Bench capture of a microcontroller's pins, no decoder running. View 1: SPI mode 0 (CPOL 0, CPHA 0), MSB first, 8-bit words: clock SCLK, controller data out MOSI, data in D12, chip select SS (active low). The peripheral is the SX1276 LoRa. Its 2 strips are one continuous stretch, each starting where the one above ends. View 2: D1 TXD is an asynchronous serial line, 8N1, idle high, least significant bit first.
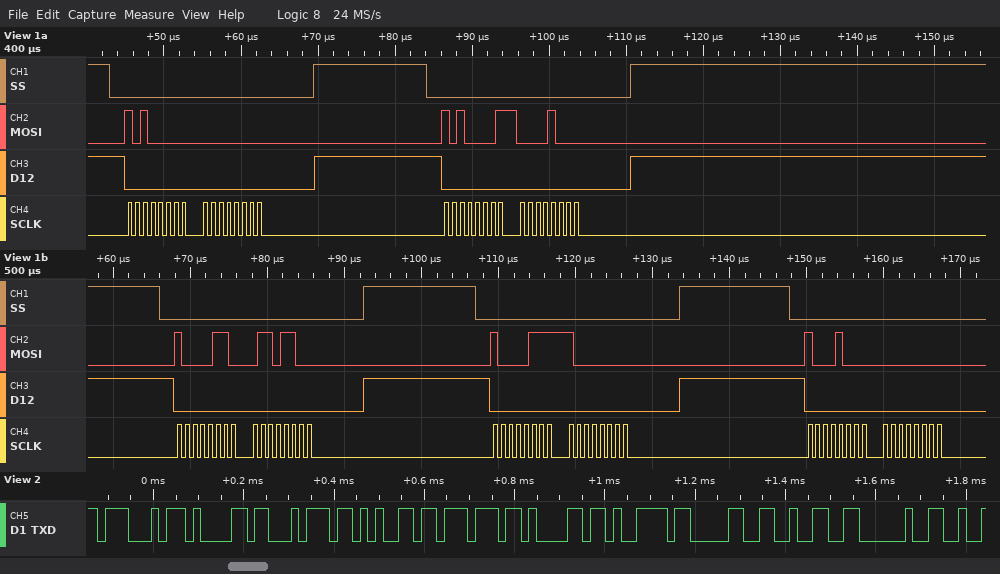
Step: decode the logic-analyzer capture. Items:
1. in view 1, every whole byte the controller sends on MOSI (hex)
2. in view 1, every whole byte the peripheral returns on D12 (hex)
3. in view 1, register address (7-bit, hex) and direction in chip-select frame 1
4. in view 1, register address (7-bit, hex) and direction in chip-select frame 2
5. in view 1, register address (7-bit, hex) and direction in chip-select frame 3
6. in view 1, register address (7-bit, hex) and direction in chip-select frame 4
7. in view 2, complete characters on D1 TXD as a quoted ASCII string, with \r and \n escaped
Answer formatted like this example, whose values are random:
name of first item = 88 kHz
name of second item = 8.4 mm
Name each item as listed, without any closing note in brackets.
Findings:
in view 1, every whole byte the controller sends on MOSI = 0xA0 0x00 0xA1 0x08 0x86 0x6C 0x87 0x80 0x88 0x00
in view 1, every whole byte the peripheral returns on D12 = 0x00 0x00 0x00 0x00 0x00 0x00 0x00 0x00 0x00 0x00
in view 1, register address (7-bit, hex) and direction in chip-select frame 1 = 0x20 write
in view 1, register address (7-bit, hex) and direction in chip-select frame 2 = 0x21 write
in view 1, register address (7-bit, hex) and direction in chip-select frame 3 = 0x06 write
in view 1, register address (7-bit, hex) and direction in chip-select frame 4 = 0x07 write
in view 2, complete characters on D1 TXD as a quoted ASCII string, with \r and \n escaped = "Gateway02 "
